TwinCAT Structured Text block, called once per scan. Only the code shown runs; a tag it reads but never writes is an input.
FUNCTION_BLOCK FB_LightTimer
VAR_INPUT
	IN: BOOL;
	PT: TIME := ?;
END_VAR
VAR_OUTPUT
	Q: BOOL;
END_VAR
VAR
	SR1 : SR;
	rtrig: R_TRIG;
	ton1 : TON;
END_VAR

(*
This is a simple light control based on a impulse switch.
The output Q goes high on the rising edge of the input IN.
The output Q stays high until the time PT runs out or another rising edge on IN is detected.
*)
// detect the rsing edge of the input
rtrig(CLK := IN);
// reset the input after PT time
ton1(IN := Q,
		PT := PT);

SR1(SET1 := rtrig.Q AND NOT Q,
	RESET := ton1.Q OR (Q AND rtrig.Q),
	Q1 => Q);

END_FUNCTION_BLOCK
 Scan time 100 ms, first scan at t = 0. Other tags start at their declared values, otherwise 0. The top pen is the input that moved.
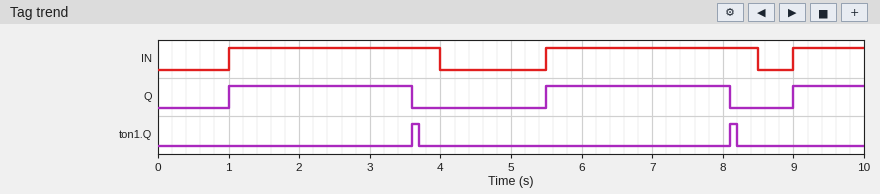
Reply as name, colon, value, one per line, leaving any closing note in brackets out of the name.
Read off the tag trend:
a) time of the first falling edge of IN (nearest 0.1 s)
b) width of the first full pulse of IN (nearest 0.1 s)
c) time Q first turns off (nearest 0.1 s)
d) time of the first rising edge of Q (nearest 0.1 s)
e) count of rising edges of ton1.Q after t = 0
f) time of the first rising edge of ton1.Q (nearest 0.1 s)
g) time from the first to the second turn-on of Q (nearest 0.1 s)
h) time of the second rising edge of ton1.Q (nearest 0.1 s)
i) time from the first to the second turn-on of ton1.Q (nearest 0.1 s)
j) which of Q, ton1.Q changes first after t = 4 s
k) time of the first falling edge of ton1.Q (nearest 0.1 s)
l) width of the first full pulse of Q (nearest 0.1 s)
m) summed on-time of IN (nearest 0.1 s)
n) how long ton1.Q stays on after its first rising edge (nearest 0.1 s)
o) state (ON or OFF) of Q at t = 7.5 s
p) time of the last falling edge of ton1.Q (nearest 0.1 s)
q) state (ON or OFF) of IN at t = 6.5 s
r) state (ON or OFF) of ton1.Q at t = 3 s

time of the first falling edge of IN: 4.0 s
width of the first full pulse of IN: 3.0 s
time Q first turns off: 3.6 s
time of the first rising edge of Q: 1.0 s
count of rising edges of ton1.Q after t = 0: 2
time of the first rising edge of ton1.Q: 3.6 s
time from the first to the second turn-on of Q: 4.5 s
time of the second rising edge of ton1.Q: 8.1 s
time from the first to the second turn-on of ton1.Q: 4.5 s
which of Q, ton1.Q changes first after t = 4 s: Q
time of the first falling edge of ton1.Q: 3.7 s
width of the first full pulse of Q: 2.6 s
summed on-time of IN: 7.0 s
how long ton1.Q stays on after its first rising edge: 0.1 s
state (ON or OFF) of Q at t = 7.5 s: ON
time of the last falling edge of ton1.Q: 8.2 s
state (ON or OFF) of IN at t = 6.5 s: ON
state (ON or OFF) of ton1.Q at t = 3 s: OFF
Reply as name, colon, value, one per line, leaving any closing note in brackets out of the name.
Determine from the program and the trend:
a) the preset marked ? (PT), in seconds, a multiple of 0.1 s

the preset marked ? (PT), in seconds, a multiple of 0.1 s: 2.5 s
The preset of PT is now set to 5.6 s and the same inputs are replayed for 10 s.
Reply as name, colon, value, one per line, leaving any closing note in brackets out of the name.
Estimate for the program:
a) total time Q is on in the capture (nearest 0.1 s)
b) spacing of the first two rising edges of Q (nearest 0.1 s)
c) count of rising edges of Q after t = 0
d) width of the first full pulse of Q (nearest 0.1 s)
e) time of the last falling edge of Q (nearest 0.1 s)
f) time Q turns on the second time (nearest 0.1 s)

total time Q is on in the capture: 5.5 s
spacing of the first two rising edges of Q: 8.0 s
count of rising edges of Q after t = 0: 2
width of the first full pulse of Q: 4.5 s
time of the last falling edge of Q: 5.5 s
time Q turns on the second time: 9.0 s
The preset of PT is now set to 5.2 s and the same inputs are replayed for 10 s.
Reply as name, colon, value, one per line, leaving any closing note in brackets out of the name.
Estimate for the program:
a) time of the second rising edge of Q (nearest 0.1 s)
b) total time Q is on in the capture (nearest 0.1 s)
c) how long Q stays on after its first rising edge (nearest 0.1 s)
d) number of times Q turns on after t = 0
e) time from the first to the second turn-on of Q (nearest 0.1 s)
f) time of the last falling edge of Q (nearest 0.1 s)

time of the second rising edge of Q: 9.0 s
total time Q is on in the capture: 5.5 s
how long Q stays on after its first rising edge: 4.5 s
number of times Q turns on after t = 0: 2
time from the first to the second turn-on of Q: 8.0 s
time of the last falling edge of Q: 5.5 s
